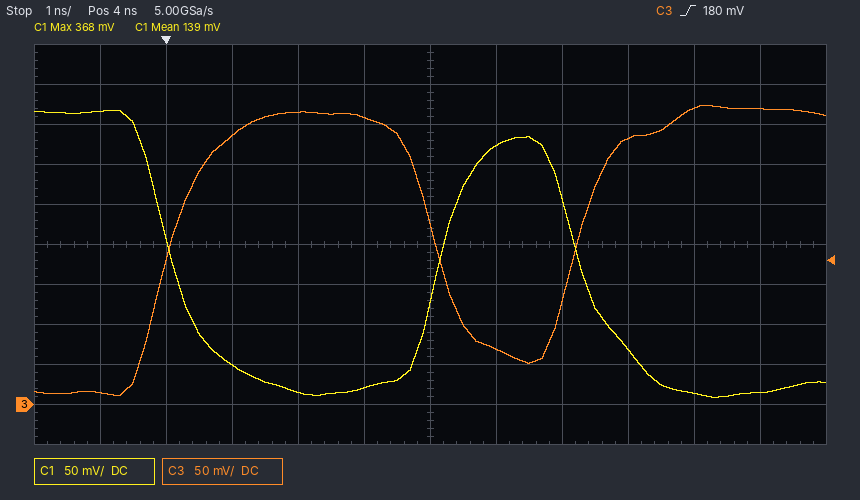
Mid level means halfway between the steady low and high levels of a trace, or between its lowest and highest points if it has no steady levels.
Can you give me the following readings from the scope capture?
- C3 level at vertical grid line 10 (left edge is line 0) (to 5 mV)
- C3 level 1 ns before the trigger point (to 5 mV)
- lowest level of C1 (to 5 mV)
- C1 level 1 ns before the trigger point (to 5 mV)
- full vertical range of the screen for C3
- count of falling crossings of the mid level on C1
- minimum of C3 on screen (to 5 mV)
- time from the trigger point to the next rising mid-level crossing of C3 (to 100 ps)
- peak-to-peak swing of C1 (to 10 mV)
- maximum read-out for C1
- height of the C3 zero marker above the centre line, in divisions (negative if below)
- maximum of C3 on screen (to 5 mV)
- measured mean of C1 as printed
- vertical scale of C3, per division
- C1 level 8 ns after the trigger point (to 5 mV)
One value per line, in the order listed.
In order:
370 mV
15 mV
10 mV
365 mV
500 mV
2
10 mV
6.2 ns
360 mV
368 mV
-4.0 div
375 mV
139 mV
50 mV
15 mV
